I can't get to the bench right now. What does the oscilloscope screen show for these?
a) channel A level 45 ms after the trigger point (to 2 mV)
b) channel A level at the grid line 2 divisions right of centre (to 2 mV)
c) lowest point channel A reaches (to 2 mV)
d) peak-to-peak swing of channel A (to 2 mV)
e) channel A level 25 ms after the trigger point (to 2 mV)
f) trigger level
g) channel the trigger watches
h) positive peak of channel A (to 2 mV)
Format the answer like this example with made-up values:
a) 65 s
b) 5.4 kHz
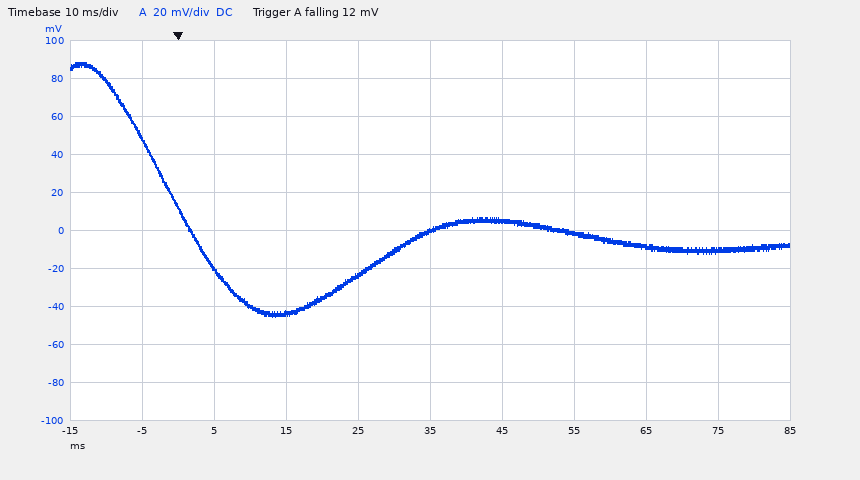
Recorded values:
a) 4 mV
b) -2 mV
c) -46 mV
d) 134 mV
e) -24 mV
f) 12 mV
g) channel A
h) 88 mV
